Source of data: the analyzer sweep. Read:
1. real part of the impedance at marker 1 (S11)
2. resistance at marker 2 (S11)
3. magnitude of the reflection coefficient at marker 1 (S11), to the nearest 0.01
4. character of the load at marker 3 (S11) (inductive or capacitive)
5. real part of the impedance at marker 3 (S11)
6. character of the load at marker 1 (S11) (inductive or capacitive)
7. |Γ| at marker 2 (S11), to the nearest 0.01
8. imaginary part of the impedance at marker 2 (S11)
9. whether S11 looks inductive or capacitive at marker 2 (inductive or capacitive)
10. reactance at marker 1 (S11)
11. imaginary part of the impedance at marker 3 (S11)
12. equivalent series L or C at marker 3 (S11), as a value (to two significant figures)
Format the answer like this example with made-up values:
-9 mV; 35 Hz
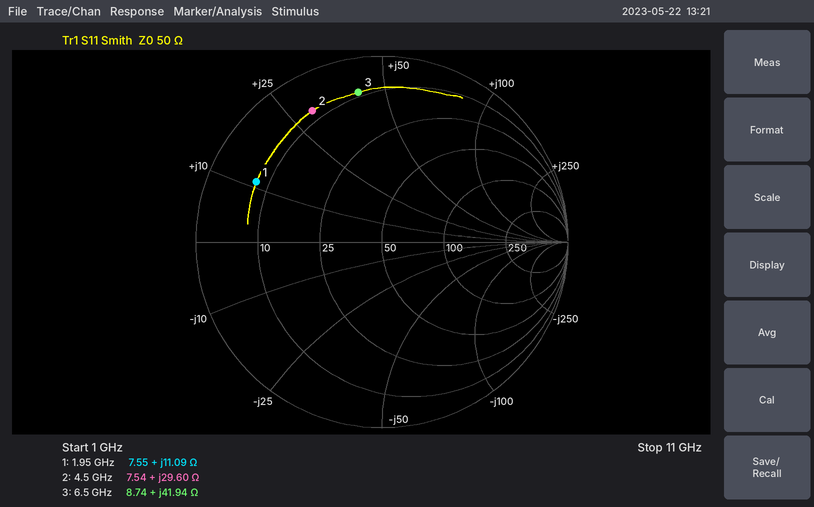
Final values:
7.55 Ω; 7.54 Ω; 0.75; inductive; 8.74 Ω; inductive; 0.80; +29.60 Ω; inductive; +11.09 Ω; +41.94 Ω; 1.0 nH
